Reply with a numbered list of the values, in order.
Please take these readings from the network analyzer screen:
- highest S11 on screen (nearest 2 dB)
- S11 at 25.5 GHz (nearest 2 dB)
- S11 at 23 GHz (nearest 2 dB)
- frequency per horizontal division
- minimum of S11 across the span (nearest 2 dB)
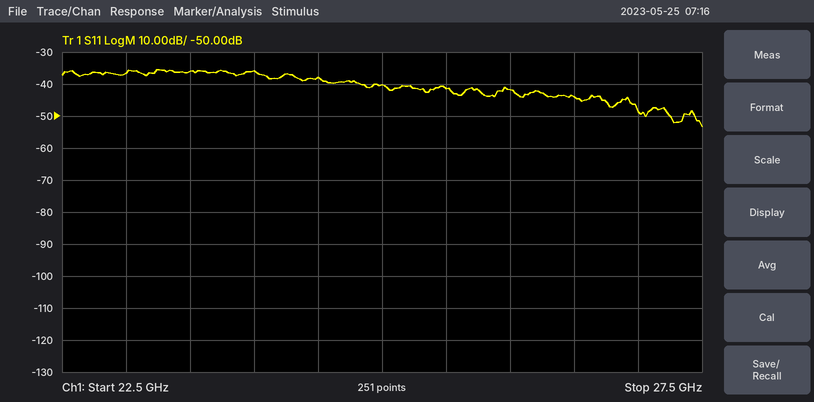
1. -36 dB
2. -42 dB
3. -36 dB
4. 500 MHz
5. -54 dB
